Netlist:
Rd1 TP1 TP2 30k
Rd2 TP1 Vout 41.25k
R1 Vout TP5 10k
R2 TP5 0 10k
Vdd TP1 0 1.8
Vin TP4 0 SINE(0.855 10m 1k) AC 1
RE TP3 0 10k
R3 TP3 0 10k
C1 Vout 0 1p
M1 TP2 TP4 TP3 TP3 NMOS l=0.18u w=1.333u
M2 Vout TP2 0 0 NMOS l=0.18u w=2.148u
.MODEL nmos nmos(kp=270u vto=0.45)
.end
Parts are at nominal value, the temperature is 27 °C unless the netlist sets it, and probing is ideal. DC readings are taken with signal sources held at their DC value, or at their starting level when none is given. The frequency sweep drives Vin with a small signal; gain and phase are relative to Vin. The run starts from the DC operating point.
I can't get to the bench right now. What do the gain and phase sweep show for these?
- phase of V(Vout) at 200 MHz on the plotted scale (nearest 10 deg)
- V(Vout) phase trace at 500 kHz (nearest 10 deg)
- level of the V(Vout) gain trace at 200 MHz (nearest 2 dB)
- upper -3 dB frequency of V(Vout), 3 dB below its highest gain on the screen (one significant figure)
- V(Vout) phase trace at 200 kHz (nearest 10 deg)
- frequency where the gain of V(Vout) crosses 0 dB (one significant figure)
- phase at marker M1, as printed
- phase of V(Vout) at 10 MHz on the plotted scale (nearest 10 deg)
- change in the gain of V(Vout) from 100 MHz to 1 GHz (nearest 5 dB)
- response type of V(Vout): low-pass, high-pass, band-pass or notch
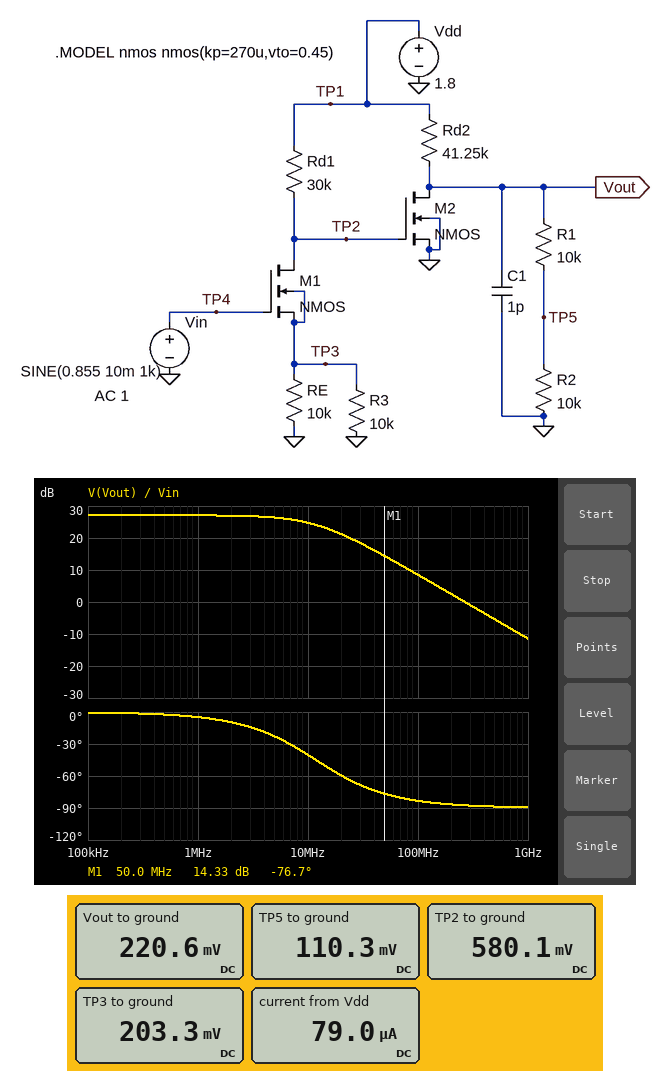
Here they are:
-90 deg
0 deg
2 dB
10 MHz
0 deg
300 MHz
-76.7 deg
-40 deg
-20 dB
low-pass
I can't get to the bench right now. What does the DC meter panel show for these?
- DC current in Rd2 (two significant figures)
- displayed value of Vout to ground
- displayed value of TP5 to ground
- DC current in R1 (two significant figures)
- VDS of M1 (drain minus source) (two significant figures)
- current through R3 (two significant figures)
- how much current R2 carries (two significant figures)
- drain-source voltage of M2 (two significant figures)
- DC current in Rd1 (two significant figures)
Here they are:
38 µA
220.6 mV
110.3 mV
11 µA
380 mV
20 µA
11 µA
220 mV
41 µA
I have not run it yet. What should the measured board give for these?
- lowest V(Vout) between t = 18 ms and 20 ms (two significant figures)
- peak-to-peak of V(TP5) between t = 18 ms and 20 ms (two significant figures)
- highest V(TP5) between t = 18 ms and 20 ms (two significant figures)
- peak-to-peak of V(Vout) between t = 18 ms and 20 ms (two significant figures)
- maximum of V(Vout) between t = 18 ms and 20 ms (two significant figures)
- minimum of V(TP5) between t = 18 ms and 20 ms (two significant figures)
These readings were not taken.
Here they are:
92 mV
160 mV
210 mV
320 mV
410 mV
46 mV
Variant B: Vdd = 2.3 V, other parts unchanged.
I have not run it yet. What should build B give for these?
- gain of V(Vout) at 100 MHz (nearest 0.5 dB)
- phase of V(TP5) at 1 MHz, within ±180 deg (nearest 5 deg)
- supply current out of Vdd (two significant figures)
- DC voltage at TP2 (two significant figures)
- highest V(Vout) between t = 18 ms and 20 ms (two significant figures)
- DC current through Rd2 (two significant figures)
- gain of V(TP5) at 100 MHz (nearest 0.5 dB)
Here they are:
-15.5 dB
0 deg
96 µA
1.1 V
29 mV
55 µA
-21.5 dB
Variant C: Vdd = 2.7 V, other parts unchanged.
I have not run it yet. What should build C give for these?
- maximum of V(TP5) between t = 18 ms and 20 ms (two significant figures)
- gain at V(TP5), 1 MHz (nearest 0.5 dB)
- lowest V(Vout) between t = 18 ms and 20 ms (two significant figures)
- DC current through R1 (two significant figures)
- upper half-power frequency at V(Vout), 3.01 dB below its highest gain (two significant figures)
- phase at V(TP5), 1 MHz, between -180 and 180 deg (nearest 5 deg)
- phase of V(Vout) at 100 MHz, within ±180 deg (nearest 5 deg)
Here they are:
10 mV
-28.5 dB
19 mV
970 nA
530 MHz
0 deg
-10 deg
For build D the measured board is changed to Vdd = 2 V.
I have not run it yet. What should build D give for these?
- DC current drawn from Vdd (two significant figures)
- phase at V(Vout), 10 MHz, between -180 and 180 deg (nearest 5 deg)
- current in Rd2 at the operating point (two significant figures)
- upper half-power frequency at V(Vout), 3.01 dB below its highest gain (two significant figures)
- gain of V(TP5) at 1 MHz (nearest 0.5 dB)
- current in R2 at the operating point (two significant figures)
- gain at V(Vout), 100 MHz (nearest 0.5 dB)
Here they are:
88 µA
-5 deg
47 µA
160 MHz
-10.5 dB
2.3 µA
-6.0 dB
